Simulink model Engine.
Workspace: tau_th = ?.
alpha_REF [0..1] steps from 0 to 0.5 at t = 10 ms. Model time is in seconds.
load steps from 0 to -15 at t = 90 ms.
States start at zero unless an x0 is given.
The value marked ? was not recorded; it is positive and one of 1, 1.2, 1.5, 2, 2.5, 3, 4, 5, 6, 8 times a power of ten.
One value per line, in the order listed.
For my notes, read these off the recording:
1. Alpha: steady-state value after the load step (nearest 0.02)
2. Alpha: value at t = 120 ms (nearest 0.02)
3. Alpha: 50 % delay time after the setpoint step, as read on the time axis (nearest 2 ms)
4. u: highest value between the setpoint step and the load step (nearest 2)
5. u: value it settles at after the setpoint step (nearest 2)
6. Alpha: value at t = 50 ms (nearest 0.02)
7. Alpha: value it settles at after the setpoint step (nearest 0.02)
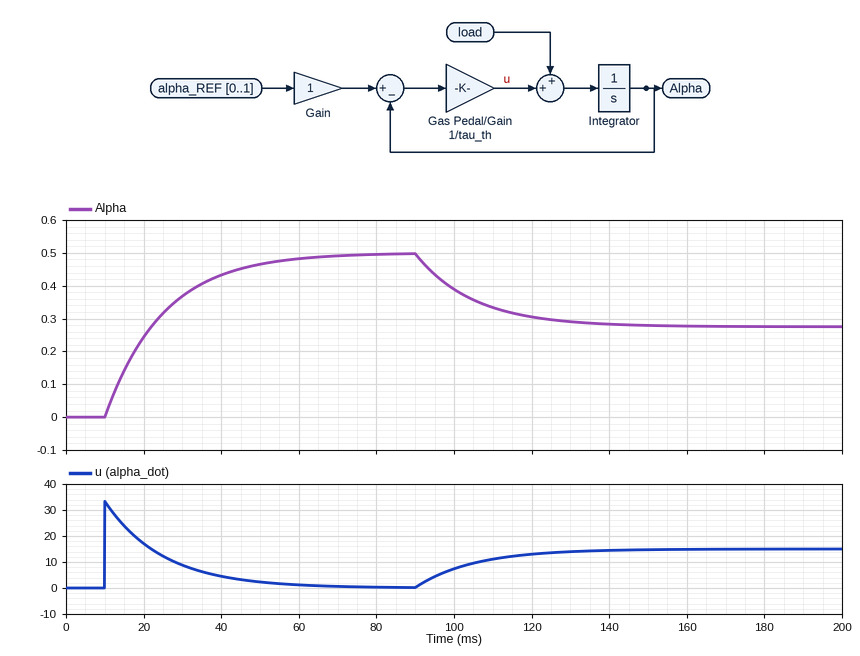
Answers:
0.28
0.30
20 ms
34
0
0.46
0.50
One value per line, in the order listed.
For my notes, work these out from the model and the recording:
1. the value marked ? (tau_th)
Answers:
0.015
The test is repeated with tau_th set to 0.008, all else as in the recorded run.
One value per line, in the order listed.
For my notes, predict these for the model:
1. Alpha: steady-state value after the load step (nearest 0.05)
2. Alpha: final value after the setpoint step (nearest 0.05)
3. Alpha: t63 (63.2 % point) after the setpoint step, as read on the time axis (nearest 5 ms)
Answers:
0.40
0.50
20 ms
